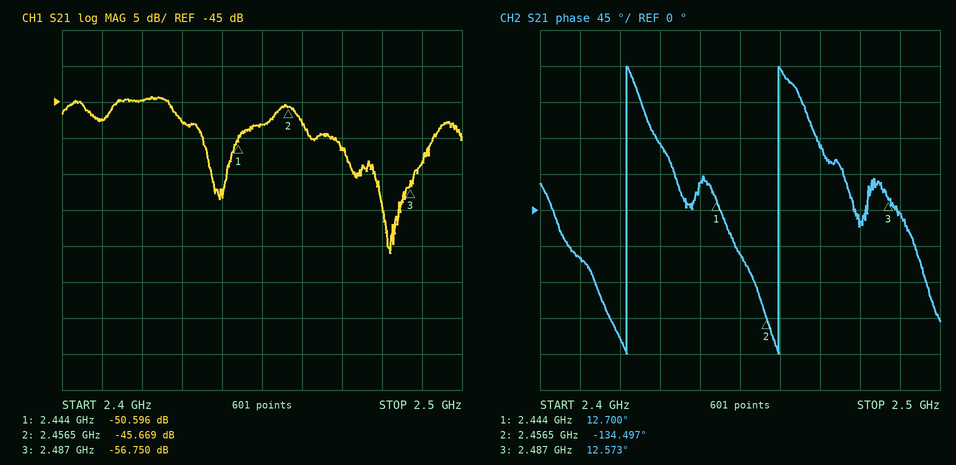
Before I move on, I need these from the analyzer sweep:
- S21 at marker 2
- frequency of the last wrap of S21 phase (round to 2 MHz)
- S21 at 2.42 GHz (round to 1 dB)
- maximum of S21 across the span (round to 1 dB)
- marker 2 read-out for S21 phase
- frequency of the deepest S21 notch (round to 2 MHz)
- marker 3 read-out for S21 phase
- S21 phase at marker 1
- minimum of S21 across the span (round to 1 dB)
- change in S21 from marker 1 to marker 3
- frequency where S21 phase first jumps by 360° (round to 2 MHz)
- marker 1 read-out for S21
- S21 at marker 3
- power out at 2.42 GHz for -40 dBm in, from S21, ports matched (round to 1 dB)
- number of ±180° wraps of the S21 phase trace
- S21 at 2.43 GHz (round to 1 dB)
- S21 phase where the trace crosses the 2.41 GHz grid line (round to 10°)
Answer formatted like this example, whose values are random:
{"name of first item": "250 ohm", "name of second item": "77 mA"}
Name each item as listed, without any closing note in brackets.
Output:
{"S21 at marker 2": "-45.669 dB", "frequency of the last wrap of S21 phase": "2.460 GHz", "S21 at 2.42 GHz": "-45 dB", "maximum of S21 across the span": "-44 dB", "marker 2 read-out for S21 phase": "-134.497°", "frequency of the deepest S21 notch": "2.482 GHz", "marker 3 read-out for S21 phase": "12.573°", "S21 phase at marker 1": "12.700°", "minimum of S21 across the span": "-66 dB", "change in S21 from marker 1 to marker 3": "-6.154 dB", "frequency where S21 phase first jumps by 360°": "2.422 GHz", "marker 1 read-out for S21": "-50.596 dB", "S21 at marker 3": "-56.750 dB", "power out at 2.42 GHz for -40 dBm in, from S21, ports matched": "-85 dBm", "number of ±180° wraps of the S21 phase trace": "2", "S21 at 2.43 GHz": "-48 dB", "S21 phase where the trace crosses the 2.41 GHz grid line": "-60°"}
